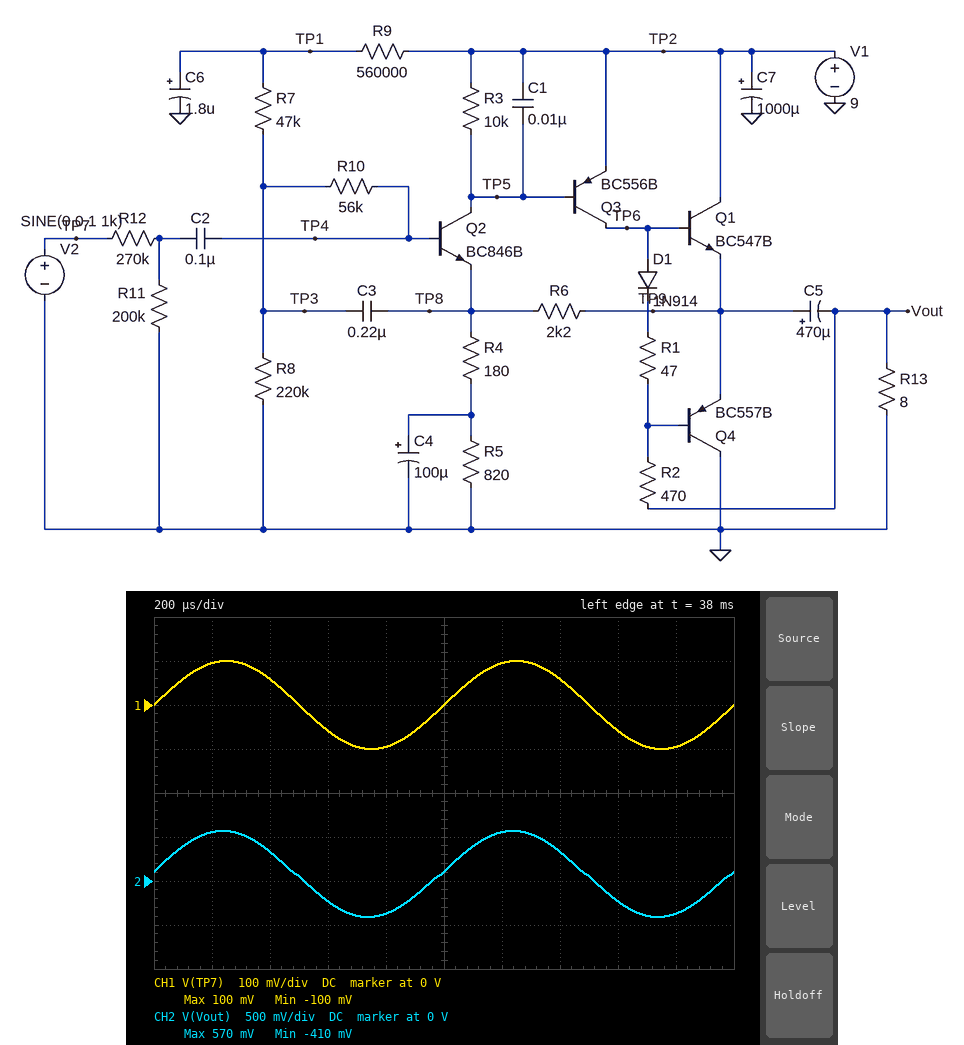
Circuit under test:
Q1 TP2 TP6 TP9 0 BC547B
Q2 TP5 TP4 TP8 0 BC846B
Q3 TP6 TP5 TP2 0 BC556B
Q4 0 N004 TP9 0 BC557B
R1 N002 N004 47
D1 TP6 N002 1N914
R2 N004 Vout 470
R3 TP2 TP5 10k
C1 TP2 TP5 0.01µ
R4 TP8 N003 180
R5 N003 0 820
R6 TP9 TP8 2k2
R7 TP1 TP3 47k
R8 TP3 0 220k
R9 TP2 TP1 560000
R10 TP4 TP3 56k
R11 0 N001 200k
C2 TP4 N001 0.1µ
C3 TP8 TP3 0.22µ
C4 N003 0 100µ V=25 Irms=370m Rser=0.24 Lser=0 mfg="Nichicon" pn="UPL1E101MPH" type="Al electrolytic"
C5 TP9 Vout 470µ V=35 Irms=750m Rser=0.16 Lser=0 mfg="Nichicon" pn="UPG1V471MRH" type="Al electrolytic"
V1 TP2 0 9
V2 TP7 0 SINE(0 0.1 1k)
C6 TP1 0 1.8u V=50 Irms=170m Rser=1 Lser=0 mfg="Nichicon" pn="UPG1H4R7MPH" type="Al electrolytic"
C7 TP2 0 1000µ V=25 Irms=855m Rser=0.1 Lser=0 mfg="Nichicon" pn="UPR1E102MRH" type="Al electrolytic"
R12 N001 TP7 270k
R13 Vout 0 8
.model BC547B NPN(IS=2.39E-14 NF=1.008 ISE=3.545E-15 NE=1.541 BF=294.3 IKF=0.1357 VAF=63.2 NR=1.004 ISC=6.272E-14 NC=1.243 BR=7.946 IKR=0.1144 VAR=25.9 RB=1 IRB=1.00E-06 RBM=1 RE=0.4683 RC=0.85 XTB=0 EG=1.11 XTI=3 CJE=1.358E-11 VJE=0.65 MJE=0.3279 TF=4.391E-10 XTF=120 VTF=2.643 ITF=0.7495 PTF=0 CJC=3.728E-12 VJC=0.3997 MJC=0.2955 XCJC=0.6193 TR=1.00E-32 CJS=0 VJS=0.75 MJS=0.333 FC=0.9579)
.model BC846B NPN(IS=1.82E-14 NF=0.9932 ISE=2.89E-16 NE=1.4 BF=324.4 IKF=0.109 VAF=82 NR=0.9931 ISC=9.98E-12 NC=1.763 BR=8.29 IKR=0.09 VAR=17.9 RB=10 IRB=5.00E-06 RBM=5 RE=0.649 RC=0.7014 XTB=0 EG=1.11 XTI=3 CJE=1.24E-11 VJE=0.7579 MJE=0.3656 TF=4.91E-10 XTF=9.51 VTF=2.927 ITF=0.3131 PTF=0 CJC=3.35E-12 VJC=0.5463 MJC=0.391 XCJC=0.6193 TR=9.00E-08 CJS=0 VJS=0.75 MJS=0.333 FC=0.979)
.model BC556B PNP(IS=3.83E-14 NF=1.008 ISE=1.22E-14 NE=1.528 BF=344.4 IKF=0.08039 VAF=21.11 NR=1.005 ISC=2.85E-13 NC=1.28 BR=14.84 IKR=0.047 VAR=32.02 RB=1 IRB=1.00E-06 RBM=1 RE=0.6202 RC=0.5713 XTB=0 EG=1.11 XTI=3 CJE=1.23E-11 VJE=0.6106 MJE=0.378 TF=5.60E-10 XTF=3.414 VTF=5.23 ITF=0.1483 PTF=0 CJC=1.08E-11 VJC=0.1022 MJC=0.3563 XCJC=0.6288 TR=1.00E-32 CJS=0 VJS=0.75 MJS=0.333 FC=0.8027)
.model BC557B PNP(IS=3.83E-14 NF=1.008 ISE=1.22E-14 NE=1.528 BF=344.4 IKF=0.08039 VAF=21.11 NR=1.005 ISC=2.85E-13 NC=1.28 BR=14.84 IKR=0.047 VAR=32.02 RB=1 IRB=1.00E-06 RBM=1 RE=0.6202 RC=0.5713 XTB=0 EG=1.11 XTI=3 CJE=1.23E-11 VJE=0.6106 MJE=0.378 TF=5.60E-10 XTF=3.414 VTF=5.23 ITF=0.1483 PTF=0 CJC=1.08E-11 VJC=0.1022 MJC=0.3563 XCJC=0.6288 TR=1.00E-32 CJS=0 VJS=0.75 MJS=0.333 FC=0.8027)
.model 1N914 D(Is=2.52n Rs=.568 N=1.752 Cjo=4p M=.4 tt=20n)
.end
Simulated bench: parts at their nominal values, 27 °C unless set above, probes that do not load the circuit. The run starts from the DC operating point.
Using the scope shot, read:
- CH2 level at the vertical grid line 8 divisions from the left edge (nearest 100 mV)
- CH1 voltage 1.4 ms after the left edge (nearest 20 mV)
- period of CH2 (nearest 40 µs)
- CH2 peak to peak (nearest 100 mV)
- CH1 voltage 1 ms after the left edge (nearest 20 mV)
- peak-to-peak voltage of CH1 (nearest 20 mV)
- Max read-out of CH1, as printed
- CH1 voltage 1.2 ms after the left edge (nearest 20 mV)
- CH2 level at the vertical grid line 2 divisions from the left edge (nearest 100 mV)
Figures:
-200 mV
60 mV
1.00 ms
1.0 V
0 V
200 mV
100 mV
100 mV
300 mV
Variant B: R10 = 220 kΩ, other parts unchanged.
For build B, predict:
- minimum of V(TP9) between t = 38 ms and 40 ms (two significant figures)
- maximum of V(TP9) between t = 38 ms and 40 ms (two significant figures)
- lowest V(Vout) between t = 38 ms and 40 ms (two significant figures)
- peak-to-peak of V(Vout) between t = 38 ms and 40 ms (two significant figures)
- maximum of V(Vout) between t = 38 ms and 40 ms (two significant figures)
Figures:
4.7 V
5.8 V
-430 mV
1.0 V
590 mV
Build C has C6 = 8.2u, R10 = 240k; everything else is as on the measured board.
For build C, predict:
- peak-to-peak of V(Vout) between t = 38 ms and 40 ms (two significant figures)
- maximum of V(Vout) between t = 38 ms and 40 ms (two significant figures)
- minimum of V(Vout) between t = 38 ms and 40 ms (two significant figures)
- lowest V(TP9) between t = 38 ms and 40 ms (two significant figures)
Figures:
1.0 V
590 mV
-430 mV
4.7 V
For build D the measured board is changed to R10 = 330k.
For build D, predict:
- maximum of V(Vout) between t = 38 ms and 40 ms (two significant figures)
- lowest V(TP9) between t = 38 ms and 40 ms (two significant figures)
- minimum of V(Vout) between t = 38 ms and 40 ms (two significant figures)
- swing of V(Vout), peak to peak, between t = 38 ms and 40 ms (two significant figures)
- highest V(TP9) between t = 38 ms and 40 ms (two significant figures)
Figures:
590 mV
4.6 V
-430 mV
1.0 V
5.7 V
